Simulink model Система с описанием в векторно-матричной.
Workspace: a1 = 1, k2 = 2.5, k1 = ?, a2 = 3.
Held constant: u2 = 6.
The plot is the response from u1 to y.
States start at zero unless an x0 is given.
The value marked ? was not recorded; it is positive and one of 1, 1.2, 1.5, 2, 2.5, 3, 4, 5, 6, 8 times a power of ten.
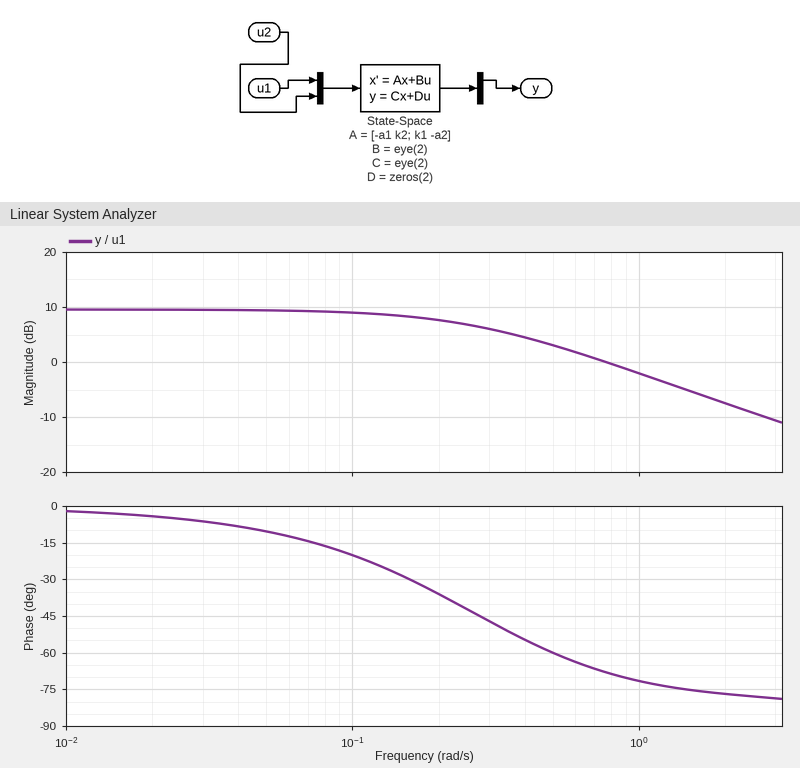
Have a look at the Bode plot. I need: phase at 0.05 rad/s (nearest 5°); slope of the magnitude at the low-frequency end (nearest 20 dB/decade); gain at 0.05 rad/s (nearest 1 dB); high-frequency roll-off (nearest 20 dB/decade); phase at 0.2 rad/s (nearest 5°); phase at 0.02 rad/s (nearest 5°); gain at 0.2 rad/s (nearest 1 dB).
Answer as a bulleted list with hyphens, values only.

- -10°
- 0 dB/decade
- 9 dB
- -20 dB/decade
- -35°
- -5°
- 8 dB
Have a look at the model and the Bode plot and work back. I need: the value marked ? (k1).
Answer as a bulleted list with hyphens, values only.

- 0.8
